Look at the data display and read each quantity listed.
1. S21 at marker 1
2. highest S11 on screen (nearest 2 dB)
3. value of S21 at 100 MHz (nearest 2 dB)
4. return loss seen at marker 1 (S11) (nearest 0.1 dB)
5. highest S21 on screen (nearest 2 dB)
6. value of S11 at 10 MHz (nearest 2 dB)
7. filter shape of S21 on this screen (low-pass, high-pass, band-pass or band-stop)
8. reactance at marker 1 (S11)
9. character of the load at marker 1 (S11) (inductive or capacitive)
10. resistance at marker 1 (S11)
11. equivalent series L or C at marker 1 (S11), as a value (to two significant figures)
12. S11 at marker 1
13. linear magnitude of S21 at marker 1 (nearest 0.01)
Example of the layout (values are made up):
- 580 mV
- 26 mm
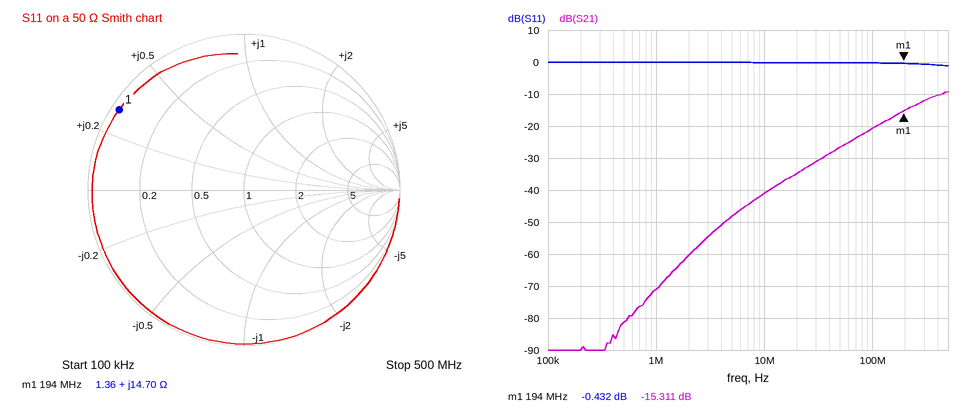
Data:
- -15.311 dB
- 0 dB
- -20 dB
- 0.4 dB
- -10 dB
- 0 dB
- high-pass
- +14.70 Ω
- inductive
- 1.36 Ω
- 12 nH
- -0.432 dB
- 0.17
